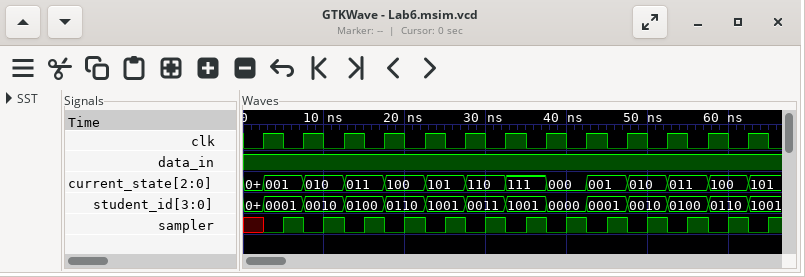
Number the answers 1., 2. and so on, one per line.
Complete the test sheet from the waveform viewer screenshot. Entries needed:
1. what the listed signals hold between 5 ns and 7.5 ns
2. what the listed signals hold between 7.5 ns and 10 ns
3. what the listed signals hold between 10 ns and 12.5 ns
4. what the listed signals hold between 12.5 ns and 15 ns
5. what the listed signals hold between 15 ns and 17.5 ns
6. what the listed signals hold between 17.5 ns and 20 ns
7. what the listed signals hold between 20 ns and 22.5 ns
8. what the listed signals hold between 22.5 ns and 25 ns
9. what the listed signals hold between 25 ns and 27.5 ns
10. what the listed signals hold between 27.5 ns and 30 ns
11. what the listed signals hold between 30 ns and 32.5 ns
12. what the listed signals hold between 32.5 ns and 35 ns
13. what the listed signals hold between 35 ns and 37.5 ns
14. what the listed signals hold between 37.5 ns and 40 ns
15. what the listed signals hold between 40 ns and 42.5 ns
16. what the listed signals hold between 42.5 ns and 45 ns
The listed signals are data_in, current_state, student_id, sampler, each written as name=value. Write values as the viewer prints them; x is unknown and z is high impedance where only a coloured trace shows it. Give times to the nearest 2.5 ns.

1. data_in=1, current_state=001, student_id=0001, sampler=1
2. data_in=1, current_state=010, student_id=0010, sampler=0
3. data_in=1, current_state=010, student_id=0010, sampler=1
4. data_in=1, current_state=011, student_id=0100, sampler=0
5. data_in=1, current_state=011, student_id=0100, sampler=1
6. data_in=1, current_state=100, student_id=0110, sampler=0
7. data_in=1, current_state=100, student_id=0110, sampler=1
8. data_in=1, current_state=101, student_id=1001, sampler=0
9. data_in=1, current_state=101, student_id=1001, sampler=1
10. data_in=1, current_state=110, student_id=0011, sampler=0
11. data_in=1, current_state=110, student_id=0011, sampler=1
12. data_in=1, current_state=111, student_id=1001, sampler=0
13. data_in=1, current_state=111, student_id=1001, sampler=1
14. data_in=1, current_state=000, student_id=0000, sampler=0
15. data_in=1, current_state=000, student_id=0000, sampler=1
16. data_in=1, current_state=001, student_id=0001, sampler=0
